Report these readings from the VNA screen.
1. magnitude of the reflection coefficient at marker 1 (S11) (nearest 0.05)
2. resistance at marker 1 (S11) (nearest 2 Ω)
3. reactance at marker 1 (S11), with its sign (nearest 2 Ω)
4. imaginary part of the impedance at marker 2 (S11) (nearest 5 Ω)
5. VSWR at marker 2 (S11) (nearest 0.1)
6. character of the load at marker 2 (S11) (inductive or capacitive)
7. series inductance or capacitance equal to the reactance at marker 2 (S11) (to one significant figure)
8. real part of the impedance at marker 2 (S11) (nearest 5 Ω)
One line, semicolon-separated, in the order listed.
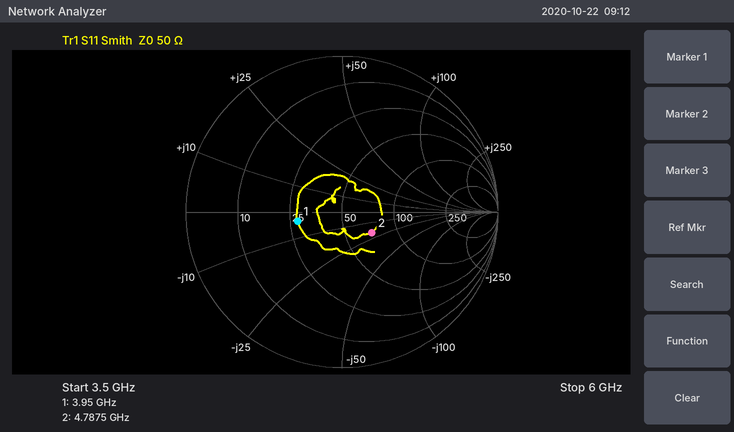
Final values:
0.30; 28 Ω; -4 Ω; -20 Ω; 1.6; capacitive; 2 pF; 70 Ω
